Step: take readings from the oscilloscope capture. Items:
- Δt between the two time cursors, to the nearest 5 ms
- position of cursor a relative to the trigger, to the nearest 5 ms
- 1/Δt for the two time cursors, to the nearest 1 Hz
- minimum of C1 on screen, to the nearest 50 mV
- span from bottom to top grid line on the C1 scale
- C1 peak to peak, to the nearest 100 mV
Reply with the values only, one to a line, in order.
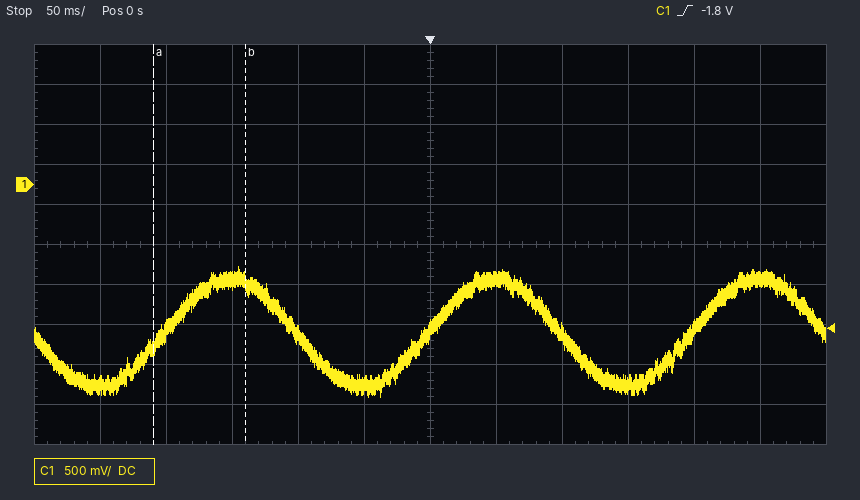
70 ms
-210 ms
14 Hz
-2.65 V
5 V
1.60 V
